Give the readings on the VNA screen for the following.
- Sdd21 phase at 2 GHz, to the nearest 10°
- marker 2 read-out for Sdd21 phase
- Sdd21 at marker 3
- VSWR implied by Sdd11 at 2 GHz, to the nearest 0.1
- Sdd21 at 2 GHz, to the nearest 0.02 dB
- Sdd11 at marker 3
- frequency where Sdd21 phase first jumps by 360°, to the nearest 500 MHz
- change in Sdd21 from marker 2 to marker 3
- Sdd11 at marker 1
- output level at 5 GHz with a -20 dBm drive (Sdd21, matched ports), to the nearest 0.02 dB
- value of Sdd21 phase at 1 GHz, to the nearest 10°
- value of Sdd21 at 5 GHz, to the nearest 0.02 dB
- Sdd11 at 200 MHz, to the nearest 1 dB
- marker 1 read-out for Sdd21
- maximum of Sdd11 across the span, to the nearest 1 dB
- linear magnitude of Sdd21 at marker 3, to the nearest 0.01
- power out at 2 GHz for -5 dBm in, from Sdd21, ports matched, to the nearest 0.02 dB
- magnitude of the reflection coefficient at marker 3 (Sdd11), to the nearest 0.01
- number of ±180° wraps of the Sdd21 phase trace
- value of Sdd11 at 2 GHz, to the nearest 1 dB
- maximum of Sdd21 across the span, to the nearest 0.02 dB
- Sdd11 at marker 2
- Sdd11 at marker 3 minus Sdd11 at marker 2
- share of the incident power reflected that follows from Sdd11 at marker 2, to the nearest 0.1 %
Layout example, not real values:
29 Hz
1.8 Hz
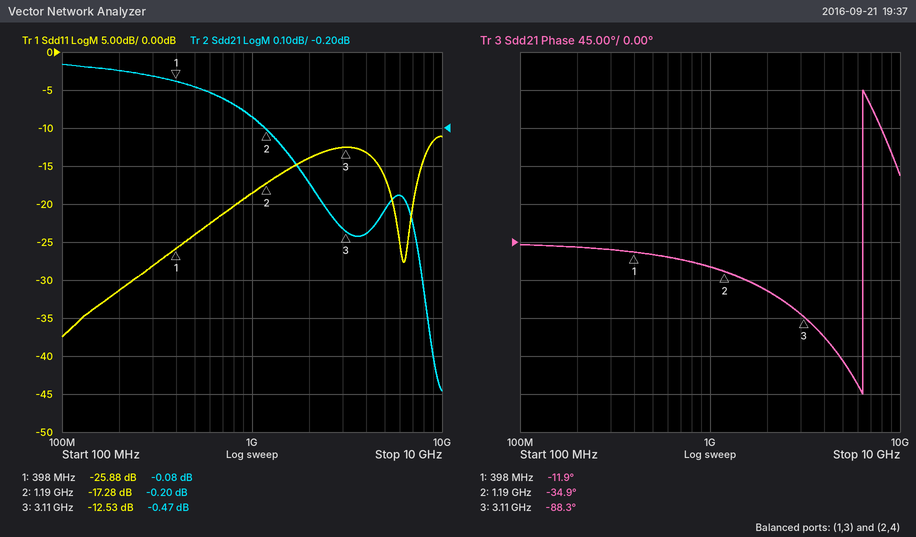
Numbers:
-60°
-34.9°
-0.47 dB
1.5
-0.34 dB
-12.53 dB
6.5 GHz
-0.27 dB
-25.88 dB
-20.42 dBm
-30°
-0.42 dB
-31 dB
-0.08 dB
-11 dB
0.95
-5.34 dBm
0.24
1
-14 dB
-0.04 dB
-17.28 dB
4.75 dB
1.9 %
